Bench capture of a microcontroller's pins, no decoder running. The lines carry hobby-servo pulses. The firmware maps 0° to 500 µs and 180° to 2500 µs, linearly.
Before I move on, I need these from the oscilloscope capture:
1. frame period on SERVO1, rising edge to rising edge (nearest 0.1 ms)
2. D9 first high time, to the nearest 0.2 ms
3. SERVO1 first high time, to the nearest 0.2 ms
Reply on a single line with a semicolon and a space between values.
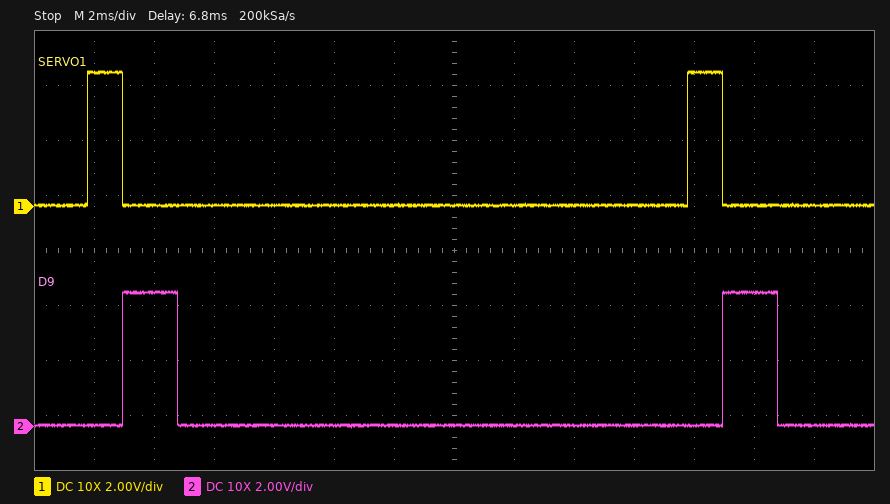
20.0 ms; 1.8 ms; 1.2 ms
